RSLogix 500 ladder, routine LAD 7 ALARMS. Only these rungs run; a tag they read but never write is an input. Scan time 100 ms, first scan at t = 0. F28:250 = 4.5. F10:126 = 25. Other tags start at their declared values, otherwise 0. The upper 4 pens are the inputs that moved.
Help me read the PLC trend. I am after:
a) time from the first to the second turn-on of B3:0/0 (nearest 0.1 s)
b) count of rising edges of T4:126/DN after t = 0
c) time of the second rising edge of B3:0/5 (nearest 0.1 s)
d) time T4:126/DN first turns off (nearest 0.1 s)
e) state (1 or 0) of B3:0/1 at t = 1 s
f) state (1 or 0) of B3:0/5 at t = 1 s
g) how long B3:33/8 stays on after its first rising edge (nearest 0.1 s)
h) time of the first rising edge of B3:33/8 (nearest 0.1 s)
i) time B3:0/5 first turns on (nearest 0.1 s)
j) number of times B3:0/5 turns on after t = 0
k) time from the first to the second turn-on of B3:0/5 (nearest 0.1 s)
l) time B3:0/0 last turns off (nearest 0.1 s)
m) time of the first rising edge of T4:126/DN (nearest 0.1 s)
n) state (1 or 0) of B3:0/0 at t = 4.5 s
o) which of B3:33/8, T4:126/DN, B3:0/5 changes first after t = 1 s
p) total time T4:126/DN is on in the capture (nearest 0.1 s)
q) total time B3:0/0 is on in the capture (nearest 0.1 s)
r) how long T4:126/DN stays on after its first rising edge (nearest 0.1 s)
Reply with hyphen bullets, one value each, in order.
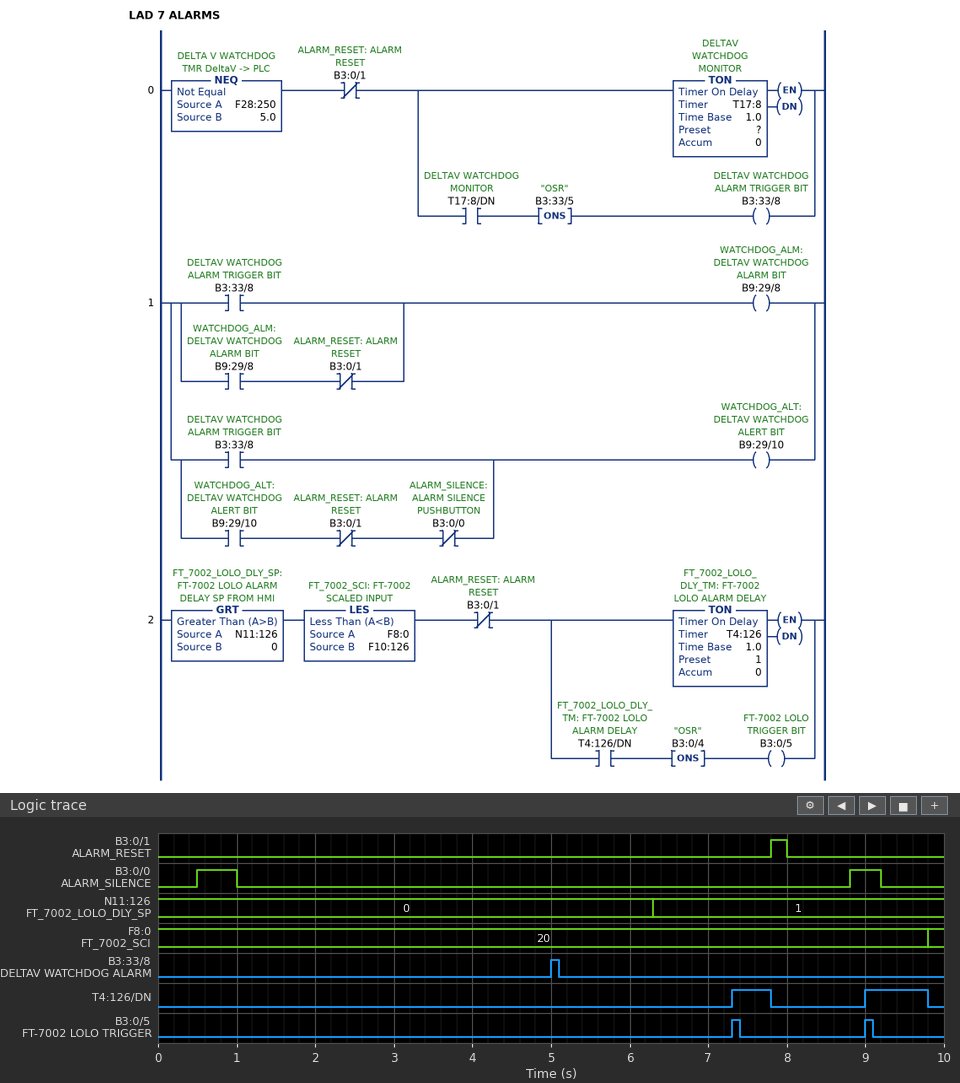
- 8.3 s
- 2
- 9.0 s
- 7.8 s
- 0
- 0
- 0.1 s
- 5.0 s
- 7.3 s
- 2
- 1.7 s
- 9.2 s
- 7.3 s
- 0
- B3:33/8
- 1.3 s
- 0.9 s
- 0.5 s
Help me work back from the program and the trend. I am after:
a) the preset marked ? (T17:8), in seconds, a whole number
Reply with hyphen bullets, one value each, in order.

- 5 s
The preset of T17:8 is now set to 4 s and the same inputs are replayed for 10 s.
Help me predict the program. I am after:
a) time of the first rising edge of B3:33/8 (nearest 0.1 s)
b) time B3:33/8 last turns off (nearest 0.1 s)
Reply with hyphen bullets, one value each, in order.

- 4.0 s
- 4.1 s
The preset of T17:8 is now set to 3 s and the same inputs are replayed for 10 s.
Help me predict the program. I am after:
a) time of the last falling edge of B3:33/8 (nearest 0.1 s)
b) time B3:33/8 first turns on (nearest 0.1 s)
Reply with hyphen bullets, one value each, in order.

- 3.1 s
- 3.0 s
